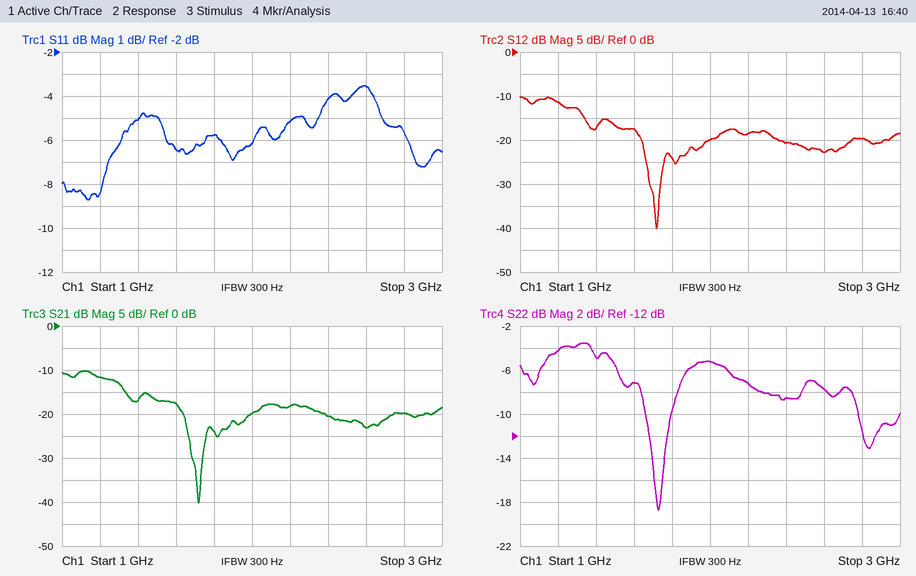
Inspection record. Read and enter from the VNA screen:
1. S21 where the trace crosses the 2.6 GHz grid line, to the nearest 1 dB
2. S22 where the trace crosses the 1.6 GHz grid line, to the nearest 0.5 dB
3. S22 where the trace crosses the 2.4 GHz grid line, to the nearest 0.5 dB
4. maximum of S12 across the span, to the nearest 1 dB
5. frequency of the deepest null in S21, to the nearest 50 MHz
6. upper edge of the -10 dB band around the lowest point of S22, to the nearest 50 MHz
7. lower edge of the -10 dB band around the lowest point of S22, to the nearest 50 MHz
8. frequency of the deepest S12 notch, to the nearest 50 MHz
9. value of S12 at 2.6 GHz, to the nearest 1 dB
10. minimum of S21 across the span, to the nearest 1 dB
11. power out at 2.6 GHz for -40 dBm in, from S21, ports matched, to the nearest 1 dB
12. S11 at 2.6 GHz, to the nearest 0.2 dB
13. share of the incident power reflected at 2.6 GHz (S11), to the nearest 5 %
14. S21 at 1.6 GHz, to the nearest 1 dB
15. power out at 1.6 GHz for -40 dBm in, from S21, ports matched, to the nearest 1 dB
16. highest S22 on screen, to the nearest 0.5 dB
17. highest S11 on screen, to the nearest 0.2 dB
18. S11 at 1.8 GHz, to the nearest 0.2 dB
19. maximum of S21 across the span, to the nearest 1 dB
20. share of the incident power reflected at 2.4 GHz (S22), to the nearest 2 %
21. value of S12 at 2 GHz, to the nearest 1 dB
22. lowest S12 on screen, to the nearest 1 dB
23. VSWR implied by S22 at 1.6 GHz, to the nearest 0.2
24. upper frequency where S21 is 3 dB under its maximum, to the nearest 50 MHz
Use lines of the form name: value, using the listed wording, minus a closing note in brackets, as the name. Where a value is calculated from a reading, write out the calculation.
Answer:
S21 where the trace crosses the 2.6 GHz grid line, to the nearest 1 dB: -23 dB
S22 where the trace crosses the 1.6 GHz grid line, to the nearest 0.5 dB: -7.0 dB
S22 where the trace crosses the 2.4 GHz grid line, to the nearest 0.5 dB: -8.5 dB
maximum of S12 across the span, to the nearest 1 dB: -10 dB
frequency of the deepest null in S21, to the nearest 50 MHz: 1.70 GHz
upper edge of the -10 dB band around the lowest point of S22, to the nearest 50 MHz: 1.80 GHz
lower edge of the -10 dB band around the lowest point of S22, to the nearest 50 MHz: 1.65 GHz
frequency of the deepest S12 notch, to the nearest 50 MHz: 1.70 GHz
value of S12 at 2.6 GHz, to the nearest 1 dB: -23 dB
minimum of S21 across the span, to the nearest 1 dB: -40 dB
power out at 2.6 GHz for -40 dBm in, from S21, ports matched, to the nearest 1 dB: -40 dBm + (-23 dB) = -63 dBm
S11 at 2.6 GHz, to the nearest 0.2 dB: -3.6 dB
share of the incident power reflected at 2.6 GHz (S11), to the nearest 5 %: 10^(-3.6/10) ≈ 43.7 %, so 45 % to the nearest 5 %
S21 at 1.6 GHz, to the nearest 1 dB: -18 dB
power out at 1.6 GHz for -40 dBm in, from S21, ports matched, to the nearest 1 dB: -40 dBm + (-18 dB) = -58 dBm
highest S22 on screen, to the nearest 0.5 dB: -3.5 dB
highest S11 on screen, to the nearest 0.2 dB: -3.6 dB
S11 at 1.8 GHz, to the nearest 0.2 dB: -5.8 dB
maximum of S21 across the span, to the nearest 1 dB: -10 dB
share of the incident power reflected at 2.4 GHz (S22), to the nearest 2 %: 10^(-8.5/10) ≈ 14 %
value of S12 at 2 GHz, to the nearest 1 dB: -20 dB
lowest S12 on screen, to the nearest 1 dB: -40 dB
VSWR implied by S22 at 1.6 GHz, to the nearest 0.2: |Γ| = 10^(-7/20) = 0.4467; VSWR = (1 + 0.4467)/(1 − 0.4467) ≈ 2.6
upper frequency where S21 is 3 dB under its maximum, to the nearest 50 MHz: 1.30 GHz
